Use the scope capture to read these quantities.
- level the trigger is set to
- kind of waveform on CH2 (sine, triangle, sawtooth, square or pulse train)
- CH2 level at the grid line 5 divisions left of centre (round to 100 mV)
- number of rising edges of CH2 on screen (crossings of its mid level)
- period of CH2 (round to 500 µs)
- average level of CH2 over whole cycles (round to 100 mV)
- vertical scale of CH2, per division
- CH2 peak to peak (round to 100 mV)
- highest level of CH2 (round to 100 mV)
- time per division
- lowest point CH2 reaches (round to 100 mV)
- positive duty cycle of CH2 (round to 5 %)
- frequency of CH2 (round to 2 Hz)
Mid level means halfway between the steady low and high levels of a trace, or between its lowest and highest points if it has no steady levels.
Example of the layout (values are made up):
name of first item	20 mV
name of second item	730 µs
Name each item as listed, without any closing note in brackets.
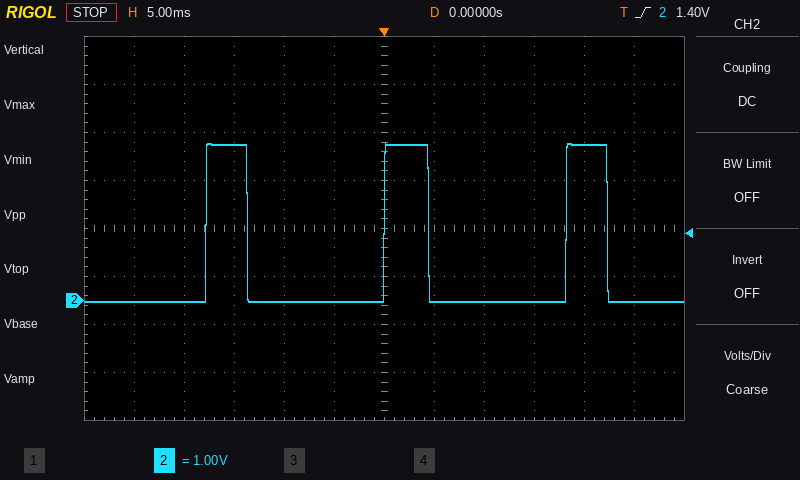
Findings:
level the trigger is set to	1.40 V
kind of waveform on CH2	pulse train
CH2 level at the grid line 5 divisions left of centre	0.0 V
number of rising edges of CH2 on screen	3
period of CH2	18.0 ms
average level of CH2 over whole cycles	800 mV
vertical scale of CH2, per division	1 V
CH2 peak to peak	3.3 V
highest level of CH2	3.3 V
time per division	5 ms
lowest point CH2 reaches	0.0 V
positive duty cycle of CH2	25 %
frequency of CH2	56 Hz
